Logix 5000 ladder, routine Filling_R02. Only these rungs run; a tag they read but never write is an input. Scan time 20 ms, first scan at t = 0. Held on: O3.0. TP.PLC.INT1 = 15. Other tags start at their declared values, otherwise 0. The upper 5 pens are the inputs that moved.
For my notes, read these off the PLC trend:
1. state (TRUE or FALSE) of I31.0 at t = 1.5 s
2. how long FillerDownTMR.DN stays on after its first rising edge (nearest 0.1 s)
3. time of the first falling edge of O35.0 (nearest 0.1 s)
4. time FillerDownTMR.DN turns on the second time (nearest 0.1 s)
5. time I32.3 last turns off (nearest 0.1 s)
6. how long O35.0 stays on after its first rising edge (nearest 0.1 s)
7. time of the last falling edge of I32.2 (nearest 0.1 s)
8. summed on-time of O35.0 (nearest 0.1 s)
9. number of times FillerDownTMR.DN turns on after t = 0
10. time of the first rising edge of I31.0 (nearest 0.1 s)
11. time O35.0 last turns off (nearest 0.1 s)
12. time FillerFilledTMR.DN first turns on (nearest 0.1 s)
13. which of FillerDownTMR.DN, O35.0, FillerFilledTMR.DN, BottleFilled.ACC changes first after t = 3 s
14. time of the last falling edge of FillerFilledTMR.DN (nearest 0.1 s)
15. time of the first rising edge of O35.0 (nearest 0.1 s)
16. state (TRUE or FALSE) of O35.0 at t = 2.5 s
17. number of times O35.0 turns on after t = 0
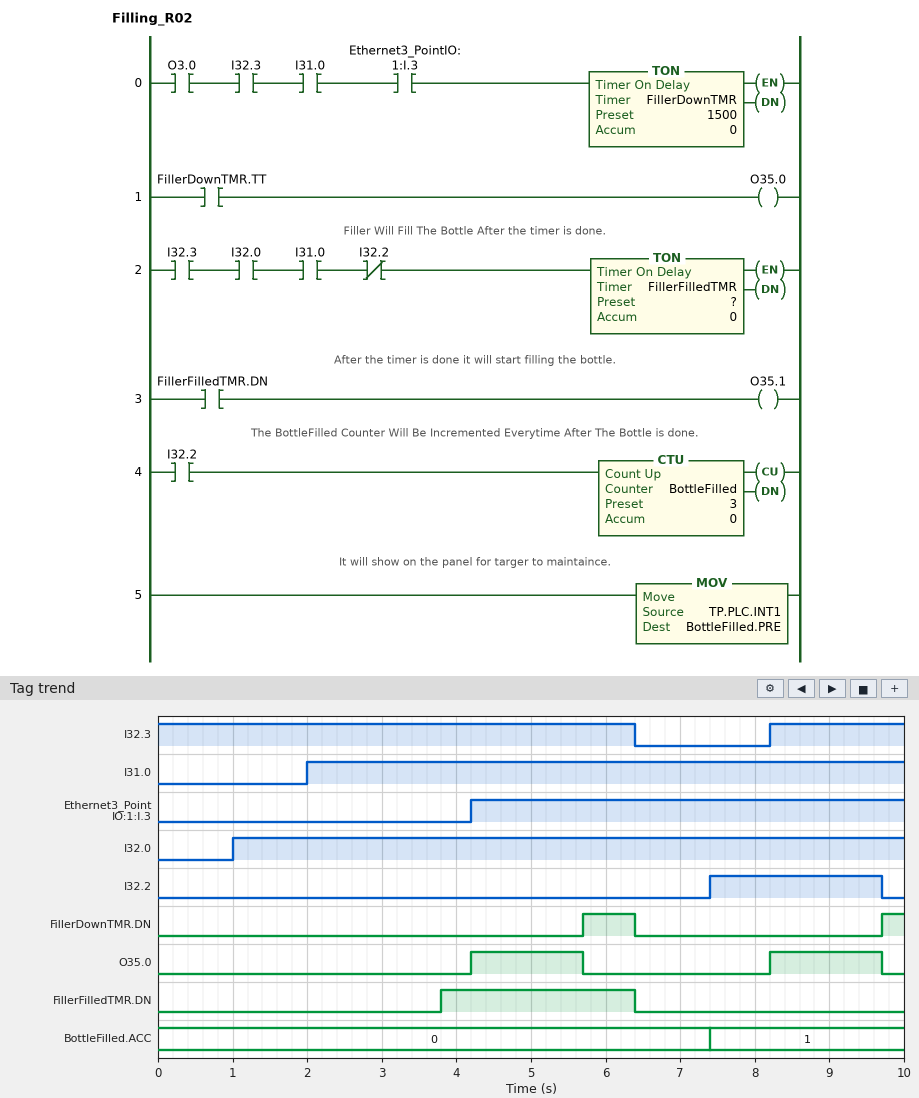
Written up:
FALSE
0.7 s
5.7 s
9.7 s
6.4 s
1.5 s
9.7 s
3.0 s
2
2.0 s
9.7 s
3.8 s
FillerFilledTMR.DN
6.4 s
4.2 s
FALSE
2
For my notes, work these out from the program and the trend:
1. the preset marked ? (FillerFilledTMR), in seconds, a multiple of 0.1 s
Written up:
1.8 s
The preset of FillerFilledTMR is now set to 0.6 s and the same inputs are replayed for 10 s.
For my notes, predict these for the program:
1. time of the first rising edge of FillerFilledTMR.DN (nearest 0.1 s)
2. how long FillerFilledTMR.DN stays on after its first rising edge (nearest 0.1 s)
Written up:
2.6 s
3.8 s
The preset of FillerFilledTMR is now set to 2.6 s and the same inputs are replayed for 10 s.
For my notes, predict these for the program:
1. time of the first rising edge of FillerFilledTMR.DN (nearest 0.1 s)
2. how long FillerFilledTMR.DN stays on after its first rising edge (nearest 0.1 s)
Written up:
4.6 s
1.8 s
